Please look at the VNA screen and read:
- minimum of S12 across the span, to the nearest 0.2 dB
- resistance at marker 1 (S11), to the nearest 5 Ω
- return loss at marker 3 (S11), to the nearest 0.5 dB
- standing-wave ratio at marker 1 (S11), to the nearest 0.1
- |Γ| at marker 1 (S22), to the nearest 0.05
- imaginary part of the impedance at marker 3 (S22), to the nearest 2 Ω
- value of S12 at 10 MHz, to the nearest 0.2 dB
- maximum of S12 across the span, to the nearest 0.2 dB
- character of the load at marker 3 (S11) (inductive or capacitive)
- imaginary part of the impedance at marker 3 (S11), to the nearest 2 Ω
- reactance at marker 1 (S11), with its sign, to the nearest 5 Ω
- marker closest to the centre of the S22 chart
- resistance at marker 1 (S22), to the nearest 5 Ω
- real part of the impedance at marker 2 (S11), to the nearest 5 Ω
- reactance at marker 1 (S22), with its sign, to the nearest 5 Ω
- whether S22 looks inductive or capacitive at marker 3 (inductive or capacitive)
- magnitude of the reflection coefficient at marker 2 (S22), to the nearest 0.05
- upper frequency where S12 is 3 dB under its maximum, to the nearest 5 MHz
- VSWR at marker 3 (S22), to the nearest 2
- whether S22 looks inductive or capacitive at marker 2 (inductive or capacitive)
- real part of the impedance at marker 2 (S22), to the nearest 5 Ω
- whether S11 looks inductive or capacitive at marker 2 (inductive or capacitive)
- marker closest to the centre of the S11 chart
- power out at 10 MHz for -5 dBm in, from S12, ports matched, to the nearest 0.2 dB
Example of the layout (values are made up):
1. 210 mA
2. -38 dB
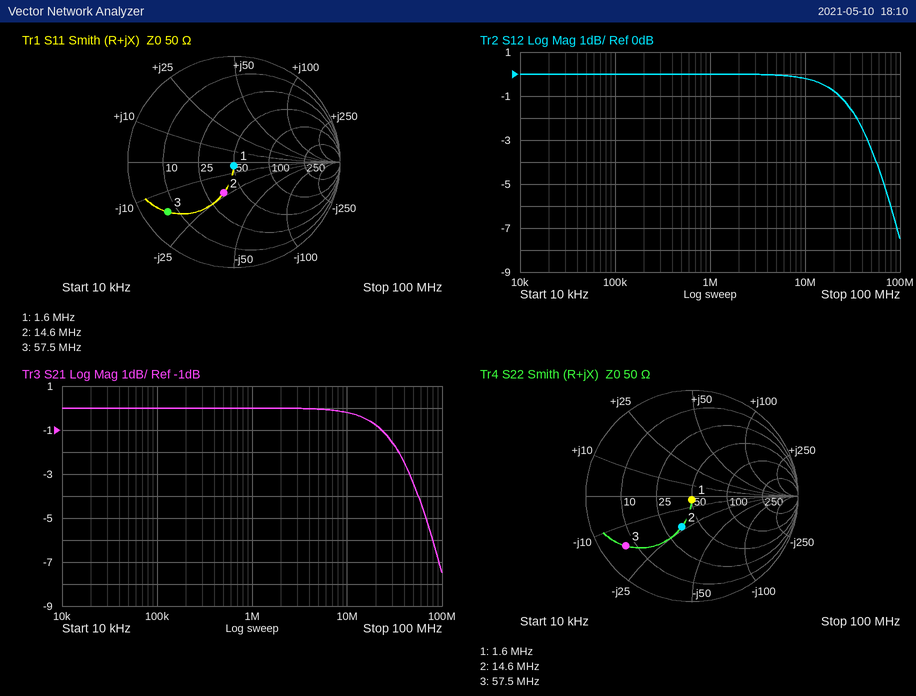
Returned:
1. -7.4 dB
2. 50 Ω
3. 2.0 dB
4. 1.1
5. 0.05
6. -16 Ω
7. -0.2 dB
8. 0.0 dB
9. capacitive
10. -16 Ω
11. -5 Ω
12. marker 1
13. 50 Ω
14. 35 Ω
15. -5 Ω
16. capacitive
17. 0.30
18. 45 MHz
19. 8
20. capacitive
21. 35 Ω
22. capacitive
23. marker 1
24. -5.2 dBm
